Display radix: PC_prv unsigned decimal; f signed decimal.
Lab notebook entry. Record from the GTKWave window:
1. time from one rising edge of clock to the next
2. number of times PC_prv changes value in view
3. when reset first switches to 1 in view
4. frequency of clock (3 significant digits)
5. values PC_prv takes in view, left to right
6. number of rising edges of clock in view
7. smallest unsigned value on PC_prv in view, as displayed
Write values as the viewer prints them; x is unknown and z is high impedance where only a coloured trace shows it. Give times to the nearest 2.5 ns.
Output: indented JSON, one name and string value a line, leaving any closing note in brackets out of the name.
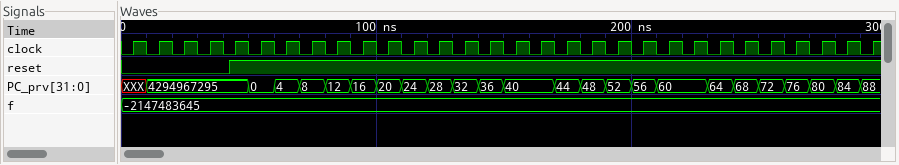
{
  "time from one rising edge of clock to the next": "10 ns",
  "number of times PC_prv changes value in view": "24",
  "when reset first switches to 1 in view": "42.5 ns",
  "frequency of clock": "100 MHz",
  "values PC_prv takes in view, left to right": "XXX, 4294967295, 0, 4, 8, 12, 16, 20, 24, 28, 32, 36, 40, 44, 48, 52, 56, 60, 64, 68, 72, 76, 80, 84, 88",
  "number of rising edges of clock in view": "30",
  "smallest unsigned value on PC_prv in view, as displayed": "0"
}
